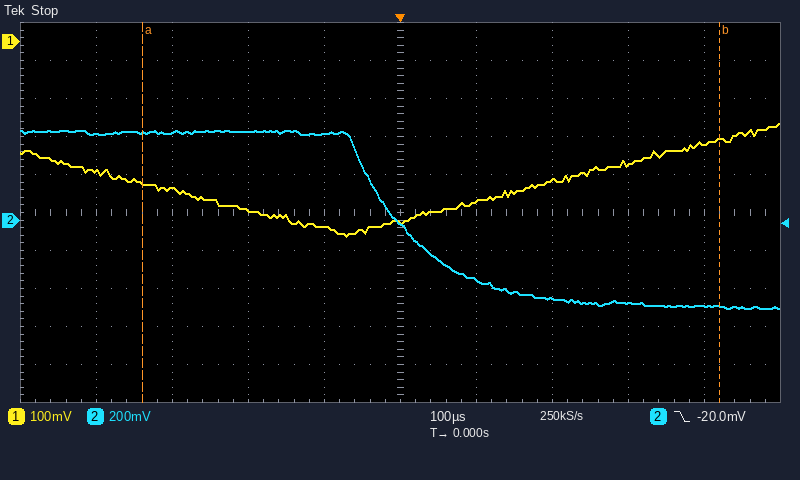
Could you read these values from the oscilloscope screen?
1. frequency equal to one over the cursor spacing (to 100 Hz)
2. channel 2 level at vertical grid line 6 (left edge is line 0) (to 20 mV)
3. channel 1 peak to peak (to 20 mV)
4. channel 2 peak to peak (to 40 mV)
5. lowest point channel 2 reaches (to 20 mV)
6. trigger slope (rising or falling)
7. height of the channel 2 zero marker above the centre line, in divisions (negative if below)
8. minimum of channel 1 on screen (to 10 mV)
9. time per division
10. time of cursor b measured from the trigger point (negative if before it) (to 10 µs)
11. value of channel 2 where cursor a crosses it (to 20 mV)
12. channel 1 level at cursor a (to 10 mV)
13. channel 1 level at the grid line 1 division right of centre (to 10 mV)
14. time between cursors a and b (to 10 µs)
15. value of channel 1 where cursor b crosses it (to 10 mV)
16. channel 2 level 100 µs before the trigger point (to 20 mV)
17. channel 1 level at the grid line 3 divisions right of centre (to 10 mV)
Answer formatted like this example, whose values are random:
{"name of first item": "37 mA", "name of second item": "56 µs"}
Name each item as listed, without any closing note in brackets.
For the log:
{"frequency equal to one over the cursor spacing": "1.3 kHz", "channel 2 level at vertical grid line 6 (left edge is line 0)": "-320 mV", "channel 1 peak to peak": "300 mV", "channel 2 peak to peak": "920 mV", "lowest point channel 2 reaches": "-460 mV", "trigger slope": "falling", "height of the channel 2 zero marker above the centre line, in divisions": "-0.2 div", "minimum of channel 1 on screen": "-510 mV", "time per division": "100 µs", "time of cursor b measured from the trigger point (negative if before it)": "+420 µs", "value of channel 2 where cursor a crosses it": "460 mV", "channel 1 level at cursor a": "-370 mV", "channel 1 level at the grid line 1 division right of centre": "-420 mV", "time between cursors a and b": "760 µs", "value of channel 1 where cursor b crosses it": "-260 mV", "channel 2 level 100 µs before the trigger point": "460 mV", "channel 1 level at the grid line 3 divisions right of centre": "-320 mV"}
